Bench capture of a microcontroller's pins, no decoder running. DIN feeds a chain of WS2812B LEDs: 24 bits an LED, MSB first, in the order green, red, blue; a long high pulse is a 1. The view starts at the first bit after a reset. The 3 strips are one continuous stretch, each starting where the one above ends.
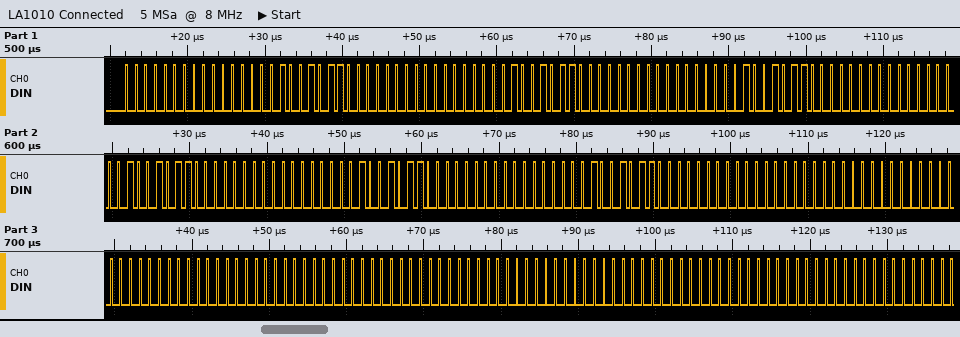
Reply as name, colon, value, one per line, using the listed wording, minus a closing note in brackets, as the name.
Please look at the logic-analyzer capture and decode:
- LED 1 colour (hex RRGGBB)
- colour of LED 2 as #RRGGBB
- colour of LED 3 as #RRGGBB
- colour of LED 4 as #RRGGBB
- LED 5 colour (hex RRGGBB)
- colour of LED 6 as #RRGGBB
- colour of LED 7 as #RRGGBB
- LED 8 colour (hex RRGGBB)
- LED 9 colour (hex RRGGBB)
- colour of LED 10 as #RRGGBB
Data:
LED 1 colour: #000096
colour of LED 2 as #RRGGBB: #000096
colour of LED 3 as #RRGGBB: #000096
colour of LED 4 as #RRGGBB: #000096
LED 5 colour: #000096
colour of LED 6 as #RRGGBB: #000096
colour of LED 7 as #RRGGBB: #000000
LED 8 colour: #000000
LED 9 colour: #000000
colour of LED 10 as #RRGGBB: #000000
